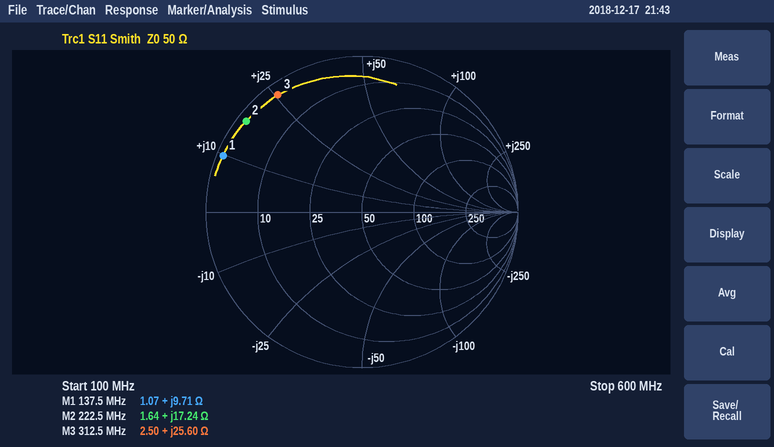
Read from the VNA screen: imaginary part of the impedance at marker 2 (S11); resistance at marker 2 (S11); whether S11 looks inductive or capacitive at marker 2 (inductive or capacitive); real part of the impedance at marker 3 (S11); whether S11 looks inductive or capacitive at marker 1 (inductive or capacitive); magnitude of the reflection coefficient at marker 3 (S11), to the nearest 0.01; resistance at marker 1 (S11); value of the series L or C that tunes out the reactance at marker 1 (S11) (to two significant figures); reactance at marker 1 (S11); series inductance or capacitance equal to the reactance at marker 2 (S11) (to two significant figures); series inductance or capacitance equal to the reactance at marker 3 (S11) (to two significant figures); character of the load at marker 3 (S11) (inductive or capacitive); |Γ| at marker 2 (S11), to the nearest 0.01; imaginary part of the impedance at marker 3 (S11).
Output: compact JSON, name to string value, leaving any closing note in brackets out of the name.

{"imaginary part of the impedance at marker 2": "+17.24 Ω", "resistance at marker 2": "1.64 Ω", "whether S11 looks inductive or capacitive at marker 2": "inductive", "real part of the impedance at marker 3": "2.50 Ω", "whether S11 looks inductive or capacitive at marker 1": "inductive", "magnitude of the reflection coefficient at marker 3 (S11), to the nearest 0.01": "0.92", "resistance at marker 1": "1.07 Ω", "value of the series L or C that tunes out the reactance at marker 1 (S11)": "120 pF", "reactance at marker 1": "+9.71 Ω", "series inductance or capacitance equal to the reactance at marker 2 (S11)": "12 nH", "series inductance or capacitance equal to the reactance at marker 3 (S11)": "13 nH", "character of the load at marker 3 (S11)": "inductive", "|Γ| at marker 2 (S11), to the nearest 0.01": "0.94", "imaginary part of the impedance at marker 3": "+25.60 Ω"}
